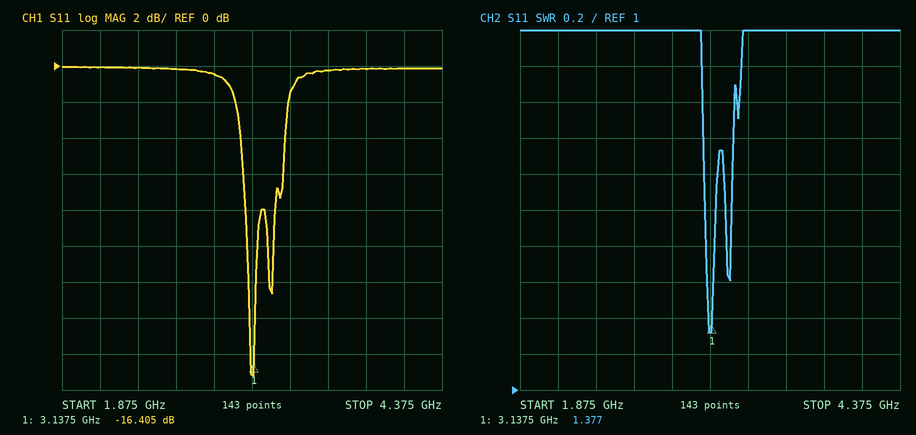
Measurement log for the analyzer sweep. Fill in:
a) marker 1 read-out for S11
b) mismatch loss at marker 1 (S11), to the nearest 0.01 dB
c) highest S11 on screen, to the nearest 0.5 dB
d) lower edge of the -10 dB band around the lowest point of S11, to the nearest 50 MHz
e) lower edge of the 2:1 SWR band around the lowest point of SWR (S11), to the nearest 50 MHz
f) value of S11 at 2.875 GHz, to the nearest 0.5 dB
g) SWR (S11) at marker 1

-16.405 dB
0.10 dB
0.0 dB
3.10 GHz
3.10 GHz
-0.5 dB
1.377
